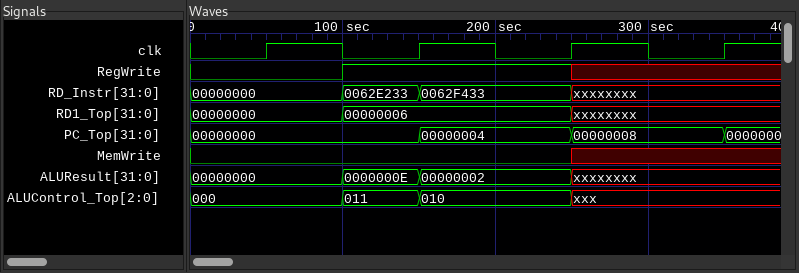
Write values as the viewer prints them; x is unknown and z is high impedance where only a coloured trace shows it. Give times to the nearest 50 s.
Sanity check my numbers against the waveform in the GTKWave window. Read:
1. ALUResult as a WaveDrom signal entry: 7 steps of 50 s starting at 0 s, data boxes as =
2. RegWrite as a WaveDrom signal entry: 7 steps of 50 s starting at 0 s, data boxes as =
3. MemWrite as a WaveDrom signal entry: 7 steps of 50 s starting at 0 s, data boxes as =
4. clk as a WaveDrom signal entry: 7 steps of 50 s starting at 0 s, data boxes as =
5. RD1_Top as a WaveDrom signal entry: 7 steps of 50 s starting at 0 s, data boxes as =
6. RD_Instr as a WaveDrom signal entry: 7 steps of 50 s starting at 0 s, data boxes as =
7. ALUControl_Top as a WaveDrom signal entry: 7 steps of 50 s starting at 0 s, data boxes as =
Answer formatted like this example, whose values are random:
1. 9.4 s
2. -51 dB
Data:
1. {name: 'ALUResult', wave: '=.==.x.', data: '00000000 0000000E 00000002'}
2. {name: 'RegWrite', wave: '0.1..x.'}
3. {name: 'MemWrite', wave: '0....x.'}
4. {name: 'clk', wave: '0101010'}
5. {name: 'RD1_Top', wave: '=.=..x.', data: '00000000 00000006'}
6. {name: 'RD_Instr', wave: '=.==.x.', data: '00000000 0062E233 0062F433'}
7. {name: 'ALUControl_Top', wave: '=.==.x.', data: '000 011 010'}
